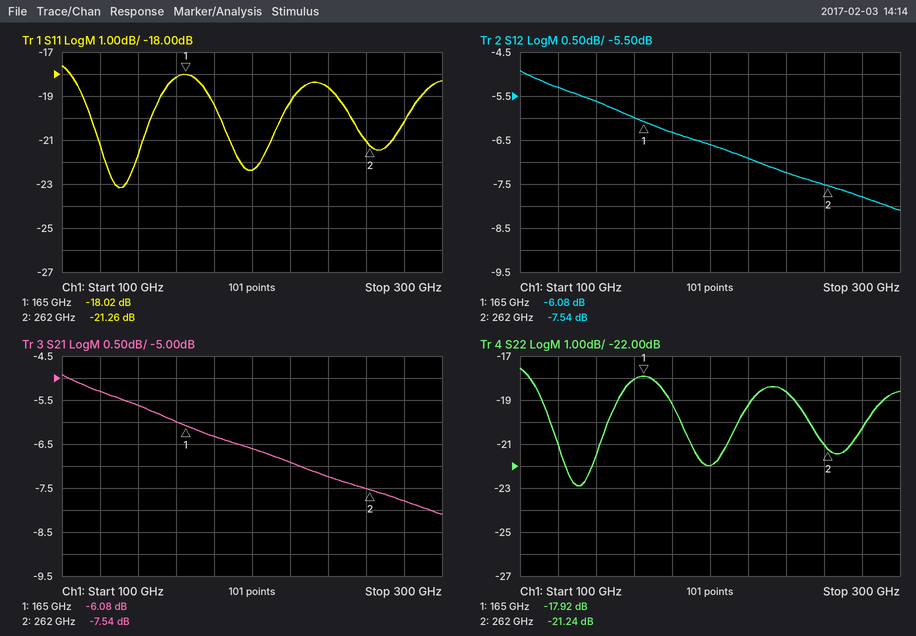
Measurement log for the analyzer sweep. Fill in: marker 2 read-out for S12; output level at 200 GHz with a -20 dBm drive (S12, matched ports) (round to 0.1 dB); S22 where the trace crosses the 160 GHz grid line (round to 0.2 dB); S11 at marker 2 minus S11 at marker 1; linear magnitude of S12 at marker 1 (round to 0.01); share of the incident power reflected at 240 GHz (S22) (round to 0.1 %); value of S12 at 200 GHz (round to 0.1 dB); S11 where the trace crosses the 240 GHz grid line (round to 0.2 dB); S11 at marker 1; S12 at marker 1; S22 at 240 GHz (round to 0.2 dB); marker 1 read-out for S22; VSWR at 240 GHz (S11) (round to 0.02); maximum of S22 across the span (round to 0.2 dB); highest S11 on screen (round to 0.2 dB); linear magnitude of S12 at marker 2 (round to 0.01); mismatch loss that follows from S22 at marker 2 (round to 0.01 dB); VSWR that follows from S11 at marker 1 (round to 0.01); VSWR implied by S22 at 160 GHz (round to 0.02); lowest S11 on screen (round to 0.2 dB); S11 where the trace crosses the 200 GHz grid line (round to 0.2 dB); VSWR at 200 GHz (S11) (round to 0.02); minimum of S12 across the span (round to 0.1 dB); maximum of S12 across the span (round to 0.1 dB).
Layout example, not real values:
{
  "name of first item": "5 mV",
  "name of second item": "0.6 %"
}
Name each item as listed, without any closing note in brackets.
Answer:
{
  "marker 2 read-out for S12": "-7.54 dB",
  "output level at 200 GHz with a -20 dBm drive (S12, matched ports)": "-26.6 dBm",
  "S22 where the trace crosses the 160 GHz grid line": "-18.0 dB",
  "S11 at marker 2 minus S11 at marker 1": "-3.24 dB",
  "linear magnitude of S12 at marker 1": "0.50",
  "share of the incident power reflected at 240 GHz (S22)": "1.4 %",
  "value of S12 at 200 GHz": "-6.6 dB",
  "S11 where the trace crosses the 240 GHz grid line": "-18.6 dB",
  "S11 at marker 1": "-18.02 dB",
  "S12 at marker 1": "-6.08 dB",
  "S22 at 240 GHz": "-18.6 dB",
  "marker 1 read-out for S22": "-17.92 dB",
  "VSWR at 240 GHz (S11)": "1.26",
  "maximum of S22 across the span": "-17.6 dB",
  "highest S11 on screen": "-17.6 dB",
  "linear magnitude of S12 at marker 2": "0.42",
  "mismatch loss that follows from S22 at marker 2": "0.03 dB",
  "VSWR that follows from S11 at marker 1": "1.29",
  "VSWR implied by S22 at 160 GHz": "1.28",
  "lowest S11 on screen": "-23.2 dB",
  "S11 where the trace crosses the 200 GHz grid line": "-22.4 dB",
  "VSWR at 200 GHz (S11)": "1.16",
  "minimum of S12 across the span": "-8.1 dB",
  "maximum of S12 across the span": "-4.9 dB"
}
